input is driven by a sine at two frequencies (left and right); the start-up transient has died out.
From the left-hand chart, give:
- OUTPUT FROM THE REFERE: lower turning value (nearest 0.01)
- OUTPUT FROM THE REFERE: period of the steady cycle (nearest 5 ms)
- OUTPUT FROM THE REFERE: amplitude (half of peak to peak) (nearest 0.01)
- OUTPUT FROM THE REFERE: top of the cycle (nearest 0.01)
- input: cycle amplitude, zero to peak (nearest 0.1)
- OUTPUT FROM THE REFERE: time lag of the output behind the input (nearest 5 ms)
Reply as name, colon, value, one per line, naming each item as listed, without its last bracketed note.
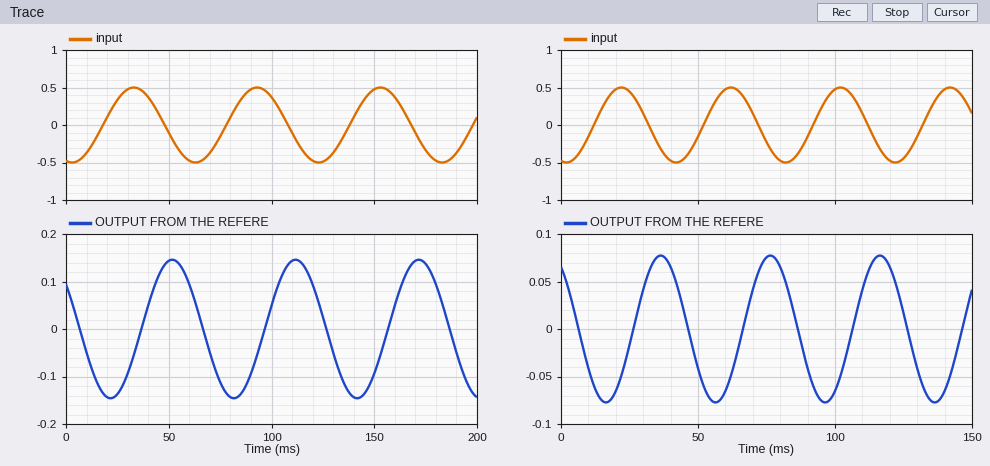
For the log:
OUTPUT FROM THE REFERE: lower turning value: -0.15
OUTPUT FROM THE REFERE: period of the steady cycle: 60 ms
OUTPUT FROM THE REFERE: amplitude (half of peak to peak): 0.15
OUTPUT FROM THE REFERE: top of the cycle: 0.15
input: cycle amplitude, zero to peak: 0.5
OUTPUT FROM THE REFERE: time lag of the output behind the input: 20 ms
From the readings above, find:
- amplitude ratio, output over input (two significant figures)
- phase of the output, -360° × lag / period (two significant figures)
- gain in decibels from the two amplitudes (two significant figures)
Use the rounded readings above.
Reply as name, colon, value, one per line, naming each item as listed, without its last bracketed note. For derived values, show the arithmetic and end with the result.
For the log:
amplitude ratio, output over input: 0.15 / 0.5 = 0.30
phase of the output, -360° × lag / period: -360 × 20 / 60 = -120°
gain in decibels from the two amplitudes: 20 log10(0.15 / 0.5) = -10 dB
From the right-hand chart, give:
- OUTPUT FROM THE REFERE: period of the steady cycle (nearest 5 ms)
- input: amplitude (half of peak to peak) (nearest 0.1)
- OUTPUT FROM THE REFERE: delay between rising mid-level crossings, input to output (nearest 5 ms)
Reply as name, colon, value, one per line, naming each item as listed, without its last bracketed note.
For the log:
OUTPUT FROM THE REFERE: period of the steady cycle: 40 ms
input: amplitude (half of peak to peak): 0.5
OUTPUT FROM THE REFERE: delay between rising mid-level crossings, input to output: 15 ms
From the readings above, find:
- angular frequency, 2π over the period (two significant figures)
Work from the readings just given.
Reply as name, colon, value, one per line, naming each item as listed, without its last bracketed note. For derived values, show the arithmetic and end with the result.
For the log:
angular frequency, 2π over the period: 2π / 40 = 0.16 rad/ms
